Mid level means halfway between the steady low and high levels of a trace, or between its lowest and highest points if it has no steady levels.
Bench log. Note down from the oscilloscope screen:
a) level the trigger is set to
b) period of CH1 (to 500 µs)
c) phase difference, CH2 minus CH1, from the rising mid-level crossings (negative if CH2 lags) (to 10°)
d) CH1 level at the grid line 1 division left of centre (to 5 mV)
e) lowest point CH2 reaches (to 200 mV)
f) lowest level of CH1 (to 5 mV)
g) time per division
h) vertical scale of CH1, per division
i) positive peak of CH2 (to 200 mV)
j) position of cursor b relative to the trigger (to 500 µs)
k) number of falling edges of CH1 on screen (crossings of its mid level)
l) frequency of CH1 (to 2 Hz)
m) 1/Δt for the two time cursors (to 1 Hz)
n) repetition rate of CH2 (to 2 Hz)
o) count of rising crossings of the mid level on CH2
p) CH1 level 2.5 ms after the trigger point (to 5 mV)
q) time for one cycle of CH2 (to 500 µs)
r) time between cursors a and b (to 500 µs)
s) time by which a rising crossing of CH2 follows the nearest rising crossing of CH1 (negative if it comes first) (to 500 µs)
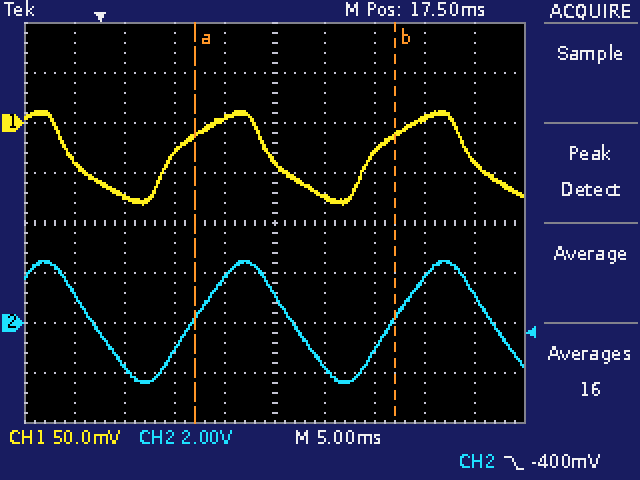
-400 mV
20.0 ms
-40°
5 mV
-2.4 V
-80 mV
5 ms
50 mV
2.4 V
+29.5 ms
3
50 Hz
50 Hz
50 Hz
2
-75 mV
20.0 ms
20.0 ms
+2.0 ms
